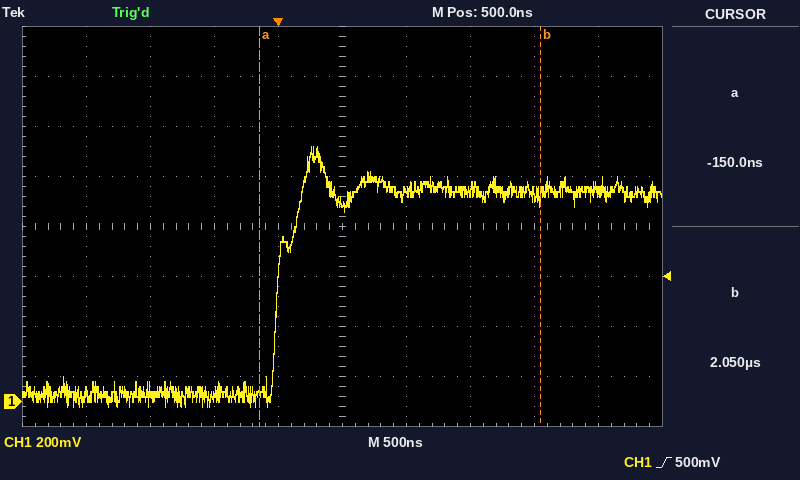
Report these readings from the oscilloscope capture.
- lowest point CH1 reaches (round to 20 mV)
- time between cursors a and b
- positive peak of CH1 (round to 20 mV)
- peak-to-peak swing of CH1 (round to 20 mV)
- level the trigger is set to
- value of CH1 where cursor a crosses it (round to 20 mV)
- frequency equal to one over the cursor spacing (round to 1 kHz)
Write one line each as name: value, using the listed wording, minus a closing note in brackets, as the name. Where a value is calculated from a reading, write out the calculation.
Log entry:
lowest point CH1 reaches: -20 mV
time between cursors a and b: 2.05 µs − (-150 ns) = 2.20 µs
positive peak of CH1: 1.02 V
peak-to-peak swing of CH1: 1.02 V − (-20 mV) = 1.04 V
level the trigger is set to: 500 mV
value of CH1 where cursor a crosses it: 40 mV
frequency equal to one over the cursor spacing: 1 / 2.20 µs ≈ 455 kHz
